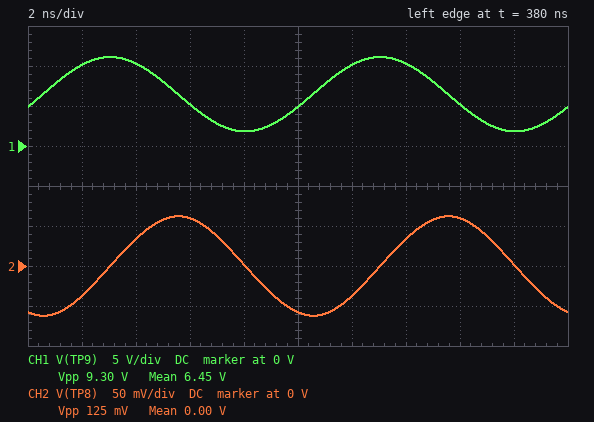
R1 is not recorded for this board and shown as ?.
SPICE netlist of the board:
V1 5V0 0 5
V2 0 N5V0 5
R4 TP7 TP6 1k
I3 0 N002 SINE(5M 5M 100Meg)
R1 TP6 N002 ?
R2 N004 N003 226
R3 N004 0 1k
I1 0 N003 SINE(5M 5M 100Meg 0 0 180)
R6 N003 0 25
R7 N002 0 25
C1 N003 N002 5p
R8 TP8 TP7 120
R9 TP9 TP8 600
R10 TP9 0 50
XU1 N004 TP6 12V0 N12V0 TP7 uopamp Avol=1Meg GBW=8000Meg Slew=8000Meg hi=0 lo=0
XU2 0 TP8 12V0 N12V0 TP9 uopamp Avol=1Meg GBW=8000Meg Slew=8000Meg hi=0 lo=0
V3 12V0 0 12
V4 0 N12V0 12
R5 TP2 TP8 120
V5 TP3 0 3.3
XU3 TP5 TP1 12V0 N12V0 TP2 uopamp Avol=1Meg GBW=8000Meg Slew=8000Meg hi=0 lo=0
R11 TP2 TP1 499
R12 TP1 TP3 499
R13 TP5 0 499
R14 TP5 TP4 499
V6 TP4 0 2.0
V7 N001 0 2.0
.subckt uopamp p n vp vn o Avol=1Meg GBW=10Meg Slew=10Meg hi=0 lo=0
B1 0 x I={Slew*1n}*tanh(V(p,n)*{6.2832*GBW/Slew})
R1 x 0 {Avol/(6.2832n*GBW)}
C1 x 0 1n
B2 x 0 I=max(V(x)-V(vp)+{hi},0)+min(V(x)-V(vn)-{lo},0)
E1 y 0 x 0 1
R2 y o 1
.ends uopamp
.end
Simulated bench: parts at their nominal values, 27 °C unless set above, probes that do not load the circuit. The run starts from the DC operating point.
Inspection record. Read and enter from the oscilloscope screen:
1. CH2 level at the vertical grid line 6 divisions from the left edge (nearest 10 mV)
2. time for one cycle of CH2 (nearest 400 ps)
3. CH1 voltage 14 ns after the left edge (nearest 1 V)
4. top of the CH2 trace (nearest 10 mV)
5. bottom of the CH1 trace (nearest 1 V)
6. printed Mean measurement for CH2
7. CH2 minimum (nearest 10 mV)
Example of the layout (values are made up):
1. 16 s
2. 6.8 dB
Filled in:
1. -40 mV
2. 10.0 ns
3. 10 V
4. 60 mV
5. 2 V
6. 0.00 V
7. -60 mV
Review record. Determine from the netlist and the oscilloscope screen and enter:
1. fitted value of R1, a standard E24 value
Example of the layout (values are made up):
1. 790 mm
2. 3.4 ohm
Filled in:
1. 240 Ω
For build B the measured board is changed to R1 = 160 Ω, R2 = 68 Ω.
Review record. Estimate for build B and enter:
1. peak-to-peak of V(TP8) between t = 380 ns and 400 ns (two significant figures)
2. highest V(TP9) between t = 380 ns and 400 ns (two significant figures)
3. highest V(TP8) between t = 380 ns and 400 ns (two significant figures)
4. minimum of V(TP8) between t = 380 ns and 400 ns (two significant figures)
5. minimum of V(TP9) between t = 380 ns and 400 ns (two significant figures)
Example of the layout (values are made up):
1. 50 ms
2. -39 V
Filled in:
1. 200 mV
2. 13 V
3. 98 mV
4. -98 mV
5. -680 mV
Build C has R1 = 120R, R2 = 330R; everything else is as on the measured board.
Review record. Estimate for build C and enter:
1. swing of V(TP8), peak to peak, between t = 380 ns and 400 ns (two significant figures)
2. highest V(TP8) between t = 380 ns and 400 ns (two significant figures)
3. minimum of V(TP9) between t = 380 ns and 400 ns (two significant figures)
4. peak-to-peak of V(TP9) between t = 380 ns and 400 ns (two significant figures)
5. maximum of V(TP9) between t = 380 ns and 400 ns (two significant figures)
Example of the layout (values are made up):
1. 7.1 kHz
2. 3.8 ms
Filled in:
1. 230 mV
2. 110 mV
3. -610 mV
4. 15 V
5. 14 V
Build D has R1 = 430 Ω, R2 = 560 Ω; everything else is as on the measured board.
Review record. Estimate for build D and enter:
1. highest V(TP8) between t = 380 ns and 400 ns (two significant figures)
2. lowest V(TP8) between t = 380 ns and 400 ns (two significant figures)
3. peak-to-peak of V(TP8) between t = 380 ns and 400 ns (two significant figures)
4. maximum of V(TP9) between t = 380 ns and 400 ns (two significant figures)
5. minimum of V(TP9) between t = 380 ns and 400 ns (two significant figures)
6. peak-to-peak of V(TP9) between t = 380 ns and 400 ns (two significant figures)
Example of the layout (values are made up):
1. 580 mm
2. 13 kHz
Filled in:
1. 33 mV
2. -33 mV
3. 67 mV
4. 9.2 V
5. 4.0 V
6. 5.2 V
